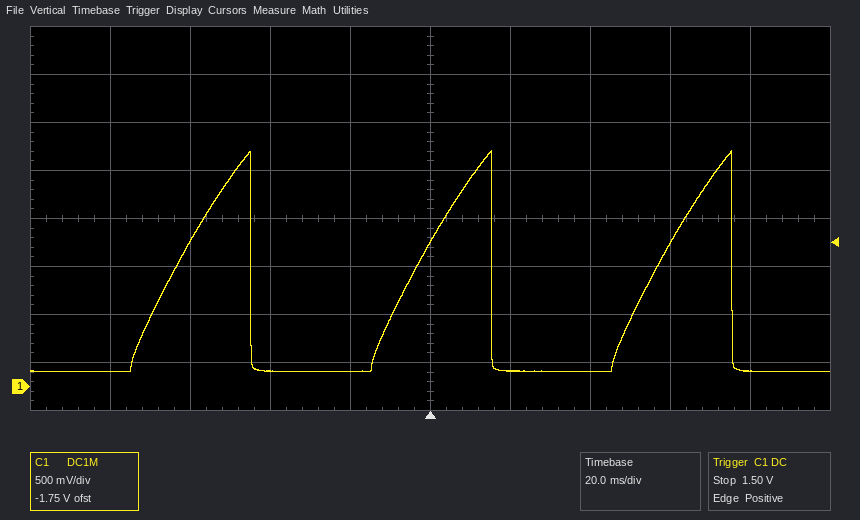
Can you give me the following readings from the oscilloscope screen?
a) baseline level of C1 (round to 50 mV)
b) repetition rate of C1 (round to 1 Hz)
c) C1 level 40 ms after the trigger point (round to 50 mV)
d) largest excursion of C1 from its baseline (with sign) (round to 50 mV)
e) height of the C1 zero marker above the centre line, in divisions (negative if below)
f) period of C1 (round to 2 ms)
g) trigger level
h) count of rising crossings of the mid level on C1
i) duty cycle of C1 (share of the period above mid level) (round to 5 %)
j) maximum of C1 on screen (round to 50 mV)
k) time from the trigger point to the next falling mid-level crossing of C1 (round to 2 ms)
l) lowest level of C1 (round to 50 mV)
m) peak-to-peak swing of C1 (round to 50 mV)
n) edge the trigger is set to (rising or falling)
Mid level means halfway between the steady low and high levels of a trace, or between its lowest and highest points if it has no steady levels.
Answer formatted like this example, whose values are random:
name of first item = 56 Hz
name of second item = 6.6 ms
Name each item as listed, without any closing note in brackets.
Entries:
baseline level of C1 = 150 mV
repetition rate of C1 = 17 Hz
C1 level 40 ms after the trigger point = 150 mV
largest excursion of C1 from its baseline (with sign) = +2.30 V
height of the C1 zero marker above the centre line, in divisions = -3.5 div
period of C1 = 60 ms
trigger level = 1.50 V
count of rising crossings of the mid level on C1 = 3
duty cycle of C1 (share of the period above mid level) = 30 %
maximum of C1 on screen = 2.45 V
time from the trigger point to the next falling mid-level crossing of C1 = 16 ms
lowest level of C1 = 150 mV
peak-to-peak swing of C1 = 2.30 V
edge the trigger is set to = rising
